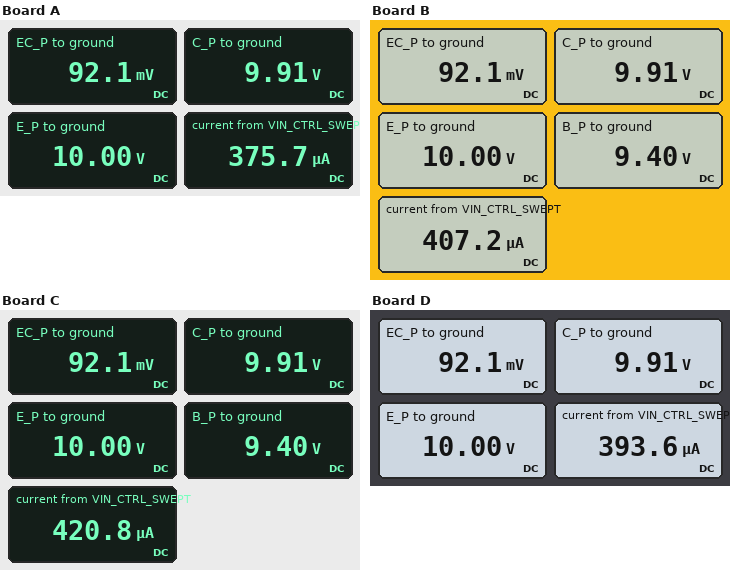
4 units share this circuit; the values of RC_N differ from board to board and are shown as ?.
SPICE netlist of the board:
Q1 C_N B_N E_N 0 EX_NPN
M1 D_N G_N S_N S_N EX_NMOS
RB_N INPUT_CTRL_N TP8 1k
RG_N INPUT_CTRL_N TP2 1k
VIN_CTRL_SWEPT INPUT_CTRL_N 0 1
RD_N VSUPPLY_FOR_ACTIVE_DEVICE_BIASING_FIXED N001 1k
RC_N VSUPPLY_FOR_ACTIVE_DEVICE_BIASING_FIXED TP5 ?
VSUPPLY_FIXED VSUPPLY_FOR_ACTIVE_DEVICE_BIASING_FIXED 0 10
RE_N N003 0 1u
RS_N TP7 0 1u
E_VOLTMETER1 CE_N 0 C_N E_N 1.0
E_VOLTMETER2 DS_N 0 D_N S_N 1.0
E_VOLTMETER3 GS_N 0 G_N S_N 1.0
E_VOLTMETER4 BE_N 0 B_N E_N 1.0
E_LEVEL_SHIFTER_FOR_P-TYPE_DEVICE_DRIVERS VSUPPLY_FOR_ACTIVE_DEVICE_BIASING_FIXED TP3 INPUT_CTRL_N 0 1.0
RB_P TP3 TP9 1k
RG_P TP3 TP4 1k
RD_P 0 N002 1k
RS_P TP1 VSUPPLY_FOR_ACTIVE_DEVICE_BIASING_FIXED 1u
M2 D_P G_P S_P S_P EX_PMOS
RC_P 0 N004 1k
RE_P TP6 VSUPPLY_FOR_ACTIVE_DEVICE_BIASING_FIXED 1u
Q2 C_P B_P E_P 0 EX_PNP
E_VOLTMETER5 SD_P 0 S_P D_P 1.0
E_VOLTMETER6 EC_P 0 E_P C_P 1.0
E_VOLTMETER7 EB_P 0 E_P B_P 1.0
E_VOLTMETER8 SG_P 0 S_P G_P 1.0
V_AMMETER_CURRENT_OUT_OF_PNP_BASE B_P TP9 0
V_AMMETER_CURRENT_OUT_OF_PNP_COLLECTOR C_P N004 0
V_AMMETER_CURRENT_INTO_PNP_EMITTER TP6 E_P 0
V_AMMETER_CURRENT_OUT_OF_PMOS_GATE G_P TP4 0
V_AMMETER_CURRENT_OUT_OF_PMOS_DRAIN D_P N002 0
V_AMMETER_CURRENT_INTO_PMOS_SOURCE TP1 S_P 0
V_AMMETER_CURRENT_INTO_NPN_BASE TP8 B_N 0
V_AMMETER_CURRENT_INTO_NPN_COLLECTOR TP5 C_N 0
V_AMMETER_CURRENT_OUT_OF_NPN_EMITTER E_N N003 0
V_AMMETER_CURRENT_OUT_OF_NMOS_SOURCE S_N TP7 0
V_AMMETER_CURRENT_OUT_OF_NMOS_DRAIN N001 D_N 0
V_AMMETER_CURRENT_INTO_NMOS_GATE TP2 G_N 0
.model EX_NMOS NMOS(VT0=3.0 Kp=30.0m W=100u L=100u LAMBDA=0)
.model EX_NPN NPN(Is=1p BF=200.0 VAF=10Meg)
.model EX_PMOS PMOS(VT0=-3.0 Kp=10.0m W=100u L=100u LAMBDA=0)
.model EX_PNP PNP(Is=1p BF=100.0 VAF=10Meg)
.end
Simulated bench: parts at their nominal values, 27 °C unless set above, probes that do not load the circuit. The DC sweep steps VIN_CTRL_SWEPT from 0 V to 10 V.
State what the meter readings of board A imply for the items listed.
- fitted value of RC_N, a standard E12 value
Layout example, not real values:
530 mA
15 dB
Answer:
330 Ω
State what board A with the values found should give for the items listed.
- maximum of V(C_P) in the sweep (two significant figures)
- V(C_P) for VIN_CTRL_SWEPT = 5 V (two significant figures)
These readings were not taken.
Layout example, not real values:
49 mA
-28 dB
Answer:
10 V
10 V
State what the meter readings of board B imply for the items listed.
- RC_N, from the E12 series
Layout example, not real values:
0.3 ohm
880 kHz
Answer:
1.2 kΩ
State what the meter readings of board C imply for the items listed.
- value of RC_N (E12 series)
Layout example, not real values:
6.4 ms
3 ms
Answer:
2.2 kΩ
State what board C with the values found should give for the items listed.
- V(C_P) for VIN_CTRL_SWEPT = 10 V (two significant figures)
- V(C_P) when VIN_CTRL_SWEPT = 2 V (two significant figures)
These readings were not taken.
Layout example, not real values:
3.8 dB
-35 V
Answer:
10 V
9.9 V
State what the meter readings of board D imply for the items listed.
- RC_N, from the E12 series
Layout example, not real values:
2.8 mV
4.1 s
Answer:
680 Ω
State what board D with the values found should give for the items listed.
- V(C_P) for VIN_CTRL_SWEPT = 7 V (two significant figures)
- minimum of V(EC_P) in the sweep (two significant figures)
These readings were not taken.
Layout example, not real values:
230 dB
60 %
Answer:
10 V
29 mV
